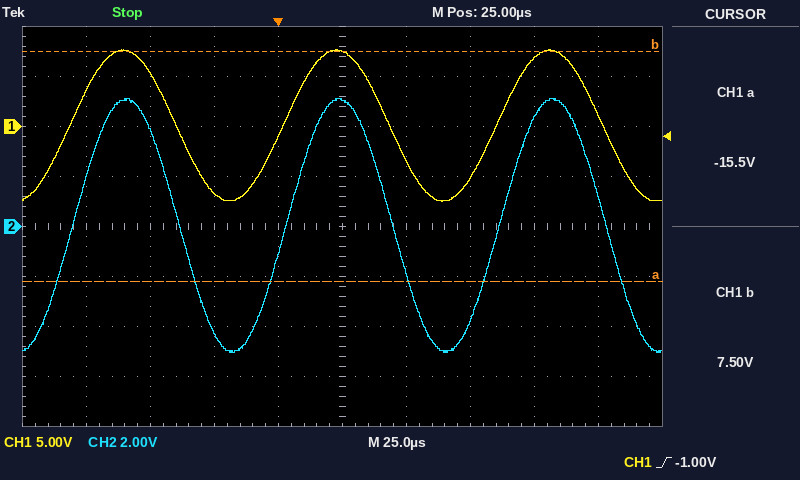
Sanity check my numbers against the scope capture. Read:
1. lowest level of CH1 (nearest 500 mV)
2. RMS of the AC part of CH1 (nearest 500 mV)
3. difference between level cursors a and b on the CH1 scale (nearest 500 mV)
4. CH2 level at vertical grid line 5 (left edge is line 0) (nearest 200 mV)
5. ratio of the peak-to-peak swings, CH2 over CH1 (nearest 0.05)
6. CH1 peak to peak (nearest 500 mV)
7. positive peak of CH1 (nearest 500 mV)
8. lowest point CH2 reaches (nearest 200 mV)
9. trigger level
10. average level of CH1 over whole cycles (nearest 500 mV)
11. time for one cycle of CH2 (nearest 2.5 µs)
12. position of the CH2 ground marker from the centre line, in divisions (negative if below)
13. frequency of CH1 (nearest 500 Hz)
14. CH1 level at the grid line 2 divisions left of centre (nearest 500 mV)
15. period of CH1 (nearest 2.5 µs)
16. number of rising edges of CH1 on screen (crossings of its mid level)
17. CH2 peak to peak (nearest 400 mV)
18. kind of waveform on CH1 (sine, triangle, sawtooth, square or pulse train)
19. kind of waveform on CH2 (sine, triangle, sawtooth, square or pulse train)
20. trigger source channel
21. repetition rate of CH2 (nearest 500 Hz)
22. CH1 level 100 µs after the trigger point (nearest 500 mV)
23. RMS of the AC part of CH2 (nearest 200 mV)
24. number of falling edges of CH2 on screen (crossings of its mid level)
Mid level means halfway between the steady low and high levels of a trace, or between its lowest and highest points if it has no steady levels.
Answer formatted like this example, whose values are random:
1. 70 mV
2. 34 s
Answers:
1. -7.5 V
2. 5.5 V
3. 23.0 V
4. 5.0 V
5. 0.65
6. 15.0 V
7. 7.5 V
8. -5.0 V
9. -1.00 V
10. 0.0 V
11. 82.5 µs
12. 0.0 div
13. 12.0 kHz
14. -6.5 V
15. 82.5 µs
16. 3
17. 10.0 V
18. sine
19. sine
20. CH1
21. 12.0 kHz
22. 7.0 V
23. 3.6 V
24. 3
